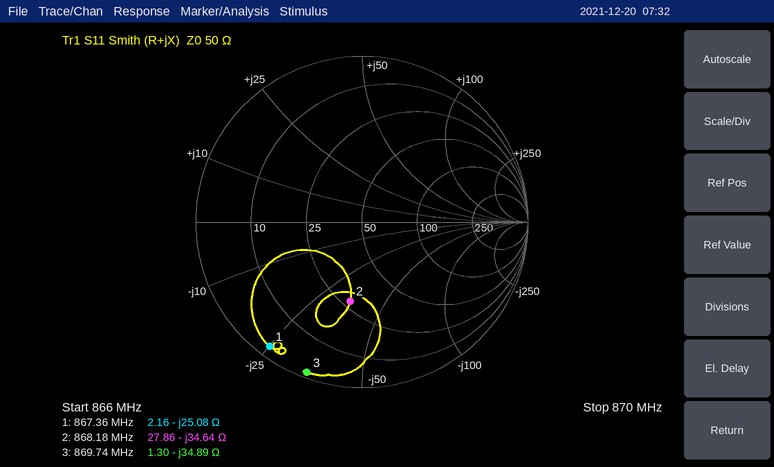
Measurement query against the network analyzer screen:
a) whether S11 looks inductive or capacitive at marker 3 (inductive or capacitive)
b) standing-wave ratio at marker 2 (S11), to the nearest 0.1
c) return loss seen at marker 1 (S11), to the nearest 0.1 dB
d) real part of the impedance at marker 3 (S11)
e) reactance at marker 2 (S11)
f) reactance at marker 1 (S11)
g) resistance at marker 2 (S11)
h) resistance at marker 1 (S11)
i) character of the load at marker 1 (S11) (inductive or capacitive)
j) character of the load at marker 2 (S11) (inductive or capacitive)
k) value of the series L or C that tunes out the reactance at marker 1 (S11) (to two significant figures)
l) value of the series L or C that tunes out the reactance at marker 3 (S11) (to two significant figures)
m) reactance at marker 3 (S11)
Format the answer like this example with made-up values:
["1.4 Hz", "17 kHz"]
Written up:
["capacitive", "2.9", "0.6 dB", "1.30 Ω", "-34.64 Ω", "-25.08 Ω", "27.86 Ω", "2.16 Ω", "capacitive", "capacitive", "4.6 nH", "6.4 nH", "-34.89 Ω"]
